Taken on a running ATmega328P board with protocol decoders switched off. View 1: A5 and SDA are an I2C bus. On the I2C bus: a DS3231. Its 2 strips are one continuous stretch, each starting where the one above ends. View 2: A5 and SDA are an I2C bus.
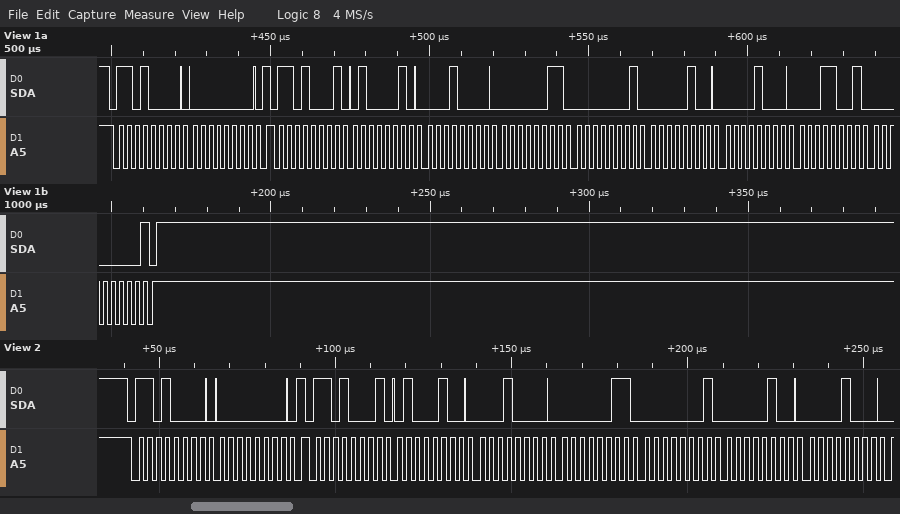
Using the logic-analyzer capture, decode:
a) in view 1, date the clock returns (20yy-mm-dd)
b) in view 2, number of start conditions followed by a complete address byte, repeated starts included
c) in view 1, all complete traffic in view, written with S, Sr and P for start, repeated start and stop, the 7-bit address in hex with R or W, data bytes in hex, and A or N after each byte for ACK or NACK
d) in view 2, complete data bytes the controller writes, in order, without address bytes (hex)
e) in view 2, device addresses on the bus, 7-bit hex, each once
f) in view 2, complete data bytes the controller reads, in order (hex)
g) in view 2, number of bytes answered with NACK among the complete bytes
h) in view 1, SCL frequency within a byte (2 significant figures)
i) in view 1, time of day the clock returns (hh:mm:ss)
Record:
2019-08-04
2
S 68W A 00 A Sr 68R A 42 A 10 A 03 A 01 A 04 A 08 A 19 A 00 N P
00
0x68
44 10 03 01 04 08
0
400 kHz
03:10:42
